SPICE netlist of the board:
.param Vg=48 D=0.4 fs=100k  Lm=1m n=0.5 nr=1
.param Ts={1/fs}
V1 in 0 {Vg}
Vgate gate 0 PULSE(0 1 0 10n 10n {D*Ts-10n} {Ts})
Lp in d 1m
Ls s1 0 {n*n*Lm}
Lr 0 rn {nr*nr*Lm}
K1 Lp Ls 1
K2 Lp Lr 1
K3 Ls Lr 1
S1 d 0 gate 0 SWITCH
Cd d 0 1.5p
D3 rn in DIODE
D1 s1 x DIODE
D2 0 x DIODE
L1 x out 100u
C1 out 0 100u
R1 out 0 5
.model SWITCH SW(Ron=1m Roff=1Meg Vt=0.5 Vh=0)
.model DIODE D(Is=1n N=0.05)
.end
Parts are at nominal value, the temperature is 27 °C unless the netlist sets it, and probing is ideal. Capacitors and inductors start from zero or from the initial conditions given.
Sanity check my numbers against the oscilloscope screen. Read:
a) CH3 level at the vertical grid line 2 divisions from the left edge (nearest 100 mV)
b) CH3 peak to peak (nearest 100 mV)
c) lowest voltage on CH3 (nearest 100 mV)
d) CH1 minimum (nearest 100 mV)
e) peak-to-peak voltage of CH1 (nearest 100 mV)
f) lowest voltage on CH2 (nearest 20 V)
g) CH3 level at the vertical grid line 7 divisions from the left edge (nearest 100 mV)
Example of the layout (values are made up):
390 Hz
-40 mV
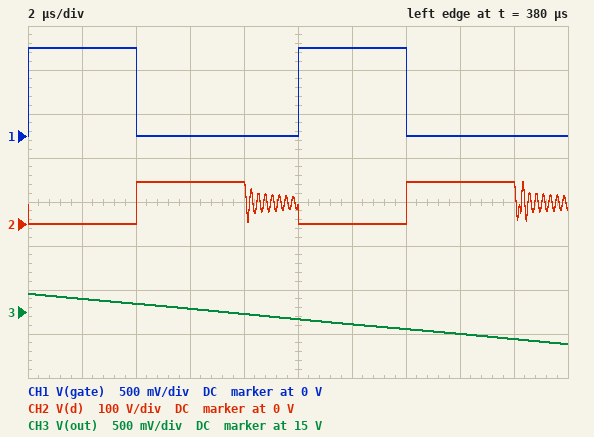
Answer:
15.1 V
600 mV
14.6 V
0 V
1.0 V
0 V
14.8 V
